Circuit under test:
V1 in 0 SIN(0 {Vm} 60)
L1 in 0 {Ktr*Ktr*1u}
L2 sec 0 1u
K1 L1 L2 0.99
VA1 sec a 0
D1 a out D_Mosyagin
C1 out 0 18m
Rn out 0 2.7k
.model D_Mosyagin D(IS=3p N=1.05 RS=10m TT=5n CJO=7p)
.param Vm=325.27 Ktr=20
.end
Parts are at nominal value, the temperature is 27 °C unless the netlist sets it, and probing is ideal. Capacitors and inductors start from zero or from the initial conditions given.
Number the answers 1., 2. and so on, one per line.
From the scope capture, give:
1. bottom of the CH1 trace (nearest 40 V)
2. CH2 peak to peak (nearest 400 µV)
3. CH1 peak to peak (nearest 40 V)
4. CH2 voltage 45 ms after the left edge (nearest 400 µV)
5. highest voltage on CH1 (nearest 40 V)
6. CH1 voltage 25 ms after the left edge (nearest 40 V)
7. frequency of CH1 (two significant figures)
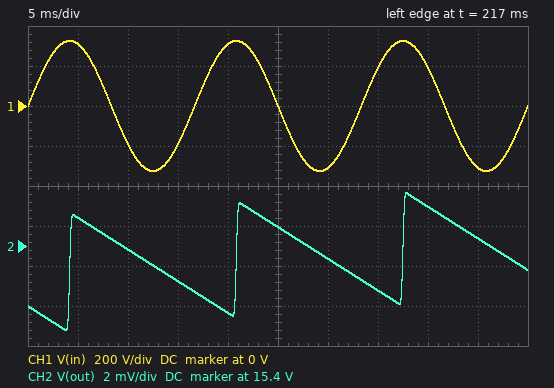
1. -320 V
2. 6.8 mV
3. 640 V
4. 15.4044 V
5. 320 V
6. 0 V
7. 60 Hz
